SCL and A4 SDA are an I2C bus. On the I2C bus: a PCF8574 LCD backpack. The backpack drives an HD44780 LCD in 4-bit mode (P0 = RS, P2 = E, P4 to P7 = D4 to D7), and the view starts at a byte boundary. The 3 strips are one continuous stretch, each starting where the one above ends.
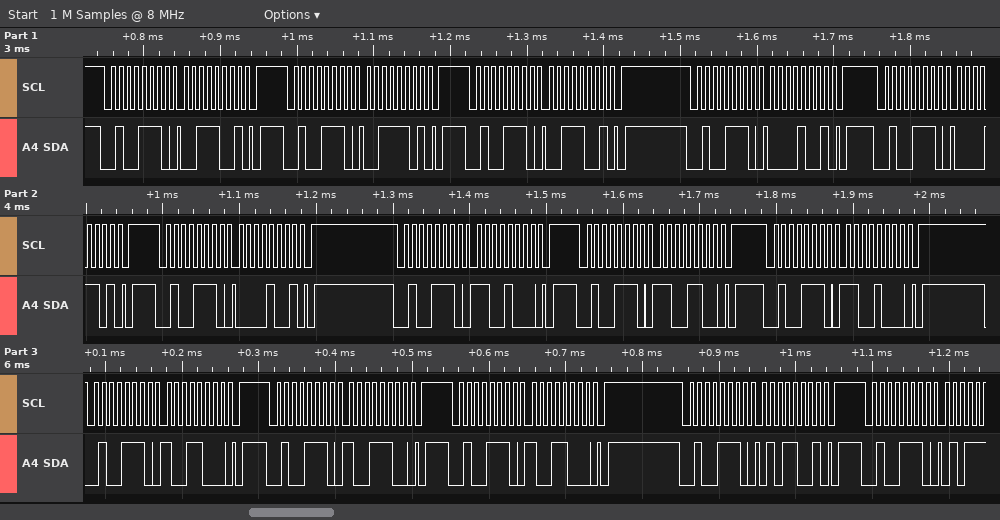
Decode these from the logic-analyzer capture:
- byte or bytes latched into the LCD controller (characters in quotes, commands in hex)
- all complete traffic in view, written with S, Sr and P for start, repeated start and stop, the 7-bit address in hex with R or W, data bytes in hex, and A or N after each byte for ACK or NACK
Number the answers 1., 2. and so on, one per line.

1. '0' 0xC9
2. S 27W A 39 A P S 27W A 3D A P S 27W A 39 A P S 27W A 09 A P S 27W A 0D A P S 27W A 09 A P S 27W A C8 A P S 27W A CC A P S 27W A C8 A P S 27W A 98 A P S 27W A 9C A P S 27W A 98 A P S 27W A 59 A P S 27W A
